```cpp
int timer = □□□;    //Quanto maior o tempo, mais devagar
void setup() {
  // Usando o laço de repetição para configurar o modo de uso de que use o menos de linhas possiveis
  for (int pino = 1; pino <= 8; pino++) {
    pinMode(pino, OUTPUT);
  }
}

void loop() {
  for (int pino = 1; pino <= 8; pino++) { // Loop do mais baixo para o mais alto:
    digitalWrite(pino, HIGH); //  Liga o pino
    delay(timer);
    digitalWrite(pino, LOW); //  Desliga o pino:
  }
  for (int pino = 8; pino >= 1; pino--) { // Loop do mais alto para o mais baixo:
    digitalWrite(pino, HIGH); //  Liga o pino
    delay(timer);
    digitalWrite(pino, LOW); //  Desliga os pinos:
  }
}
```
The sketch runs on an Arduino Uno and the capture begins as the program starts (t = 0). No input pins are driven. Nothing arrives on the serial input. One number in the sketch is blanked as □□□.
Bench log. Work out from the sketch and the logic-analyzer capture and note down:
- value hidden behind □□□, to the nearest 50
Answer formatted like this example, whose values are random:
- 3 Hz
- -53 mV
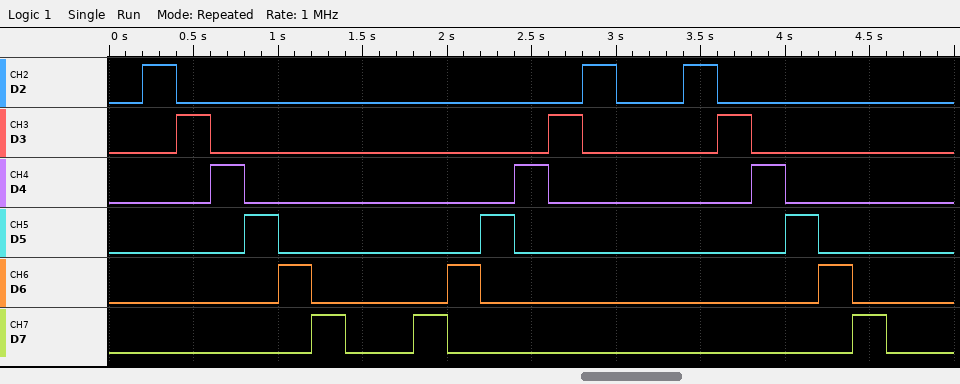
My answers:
- 200
